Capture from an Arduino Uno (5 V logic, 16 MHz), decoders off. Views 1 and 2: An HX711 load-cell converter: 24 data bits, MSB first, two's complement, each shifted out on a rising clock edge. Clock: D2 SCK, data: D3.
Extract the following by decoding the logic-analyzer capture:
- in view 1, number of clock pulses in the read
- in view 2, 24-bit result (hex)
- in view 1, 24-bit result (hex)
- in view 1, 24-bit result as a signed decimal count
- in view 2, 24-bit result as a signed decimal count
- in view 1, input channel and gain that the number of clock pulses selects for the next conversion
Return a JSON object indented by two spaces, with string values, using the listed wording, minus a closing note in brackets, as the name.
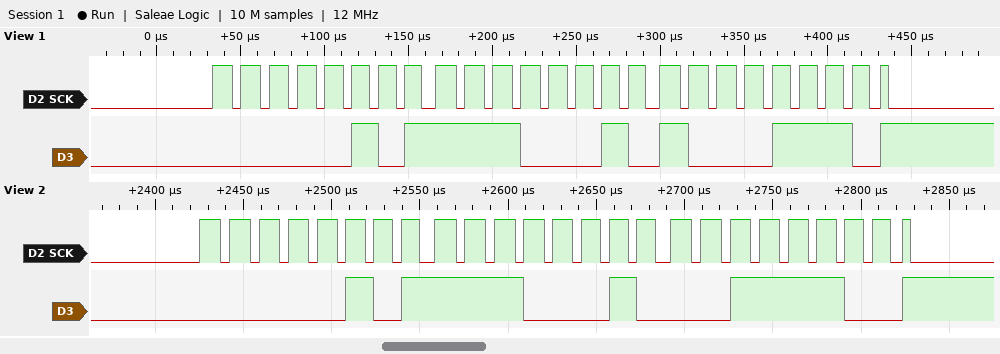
{
  "in view 1, number of clock pulses in the read": "25",
  "in view 2, 24-bit result": "0x05E23C",
  "in view 1, 24-bit result": "0x05E28E",
  "in view 1, 24-bit result as a signed decimal count": "385678",
  "in view 2, 24-bit result as a signed decimal count": "385596",
  "in view 1, input channel and gain that the number of clock pulses selects for the next conversion": "channel A, gain 128"
}
